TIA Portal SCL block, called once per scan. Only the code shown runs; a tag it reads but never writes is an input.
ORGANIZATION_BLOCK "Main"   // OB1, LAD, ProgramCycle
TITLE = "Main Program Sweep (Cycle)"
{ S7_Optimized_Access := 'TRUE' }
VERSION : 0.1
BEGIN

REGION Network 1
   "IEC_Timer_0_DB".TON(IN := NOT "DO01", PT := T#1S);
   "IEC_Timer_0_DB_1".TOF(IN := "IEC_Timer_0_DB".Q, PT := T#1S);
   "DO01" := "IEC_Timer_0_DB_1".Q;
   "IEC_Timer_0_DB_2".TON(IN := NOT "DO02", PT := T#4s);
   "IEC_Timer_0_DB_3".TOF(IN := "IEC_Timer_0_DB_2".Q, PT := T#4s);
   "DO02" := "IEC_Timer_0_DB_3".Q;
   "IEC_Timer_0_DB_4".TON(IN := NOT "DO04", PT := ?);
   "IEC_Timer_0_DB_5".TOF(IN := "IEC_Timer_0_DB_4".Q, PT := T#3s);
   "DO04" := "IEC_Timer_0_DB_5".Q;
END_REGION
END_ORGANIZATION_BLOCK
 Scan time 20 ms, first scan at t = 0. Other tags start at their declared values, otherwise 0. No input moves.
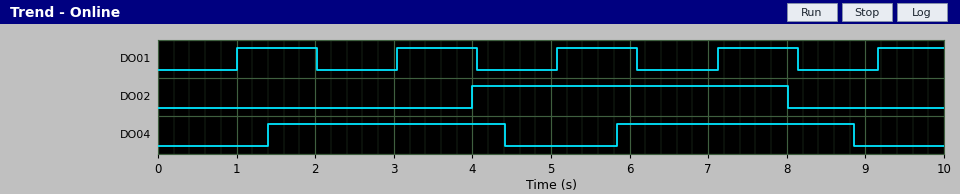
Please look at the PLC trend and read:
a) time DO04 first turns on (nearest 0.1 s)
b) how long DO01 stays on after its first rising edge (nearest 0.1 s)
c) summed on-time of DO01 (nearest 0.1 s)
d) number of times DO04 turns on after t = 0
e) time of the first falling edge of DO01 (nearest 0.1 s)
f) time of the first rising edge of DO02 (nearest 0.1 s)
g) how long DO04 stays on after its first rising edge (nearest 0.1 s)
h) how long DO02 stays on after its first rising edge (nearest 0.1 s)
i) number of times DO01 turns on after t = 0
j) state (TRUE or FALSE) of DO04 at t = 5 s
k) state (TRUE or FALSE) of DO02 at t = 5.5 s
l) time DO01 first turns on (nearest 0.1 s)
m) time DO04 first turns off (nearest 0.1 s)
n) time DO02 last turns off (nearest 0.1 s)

1.4 s
1.0 s
4.9 s
2
2.0 s
4.0 s
3.0 s
4.0 s
5
FALSE
TRUE
1.0 s
4.4 s
8.0 s
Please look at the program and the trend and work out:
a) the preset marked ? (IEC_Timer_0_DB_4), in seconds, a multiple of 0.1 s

1.4 s
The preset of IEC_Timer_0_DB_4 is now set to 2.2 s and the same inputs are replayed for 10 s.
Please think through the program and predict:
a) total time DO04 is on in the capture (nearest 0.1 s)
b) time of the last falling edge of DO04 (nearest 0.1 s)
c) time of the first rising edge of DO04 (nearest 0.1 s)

5.6 s
5.2 s
2.2 s
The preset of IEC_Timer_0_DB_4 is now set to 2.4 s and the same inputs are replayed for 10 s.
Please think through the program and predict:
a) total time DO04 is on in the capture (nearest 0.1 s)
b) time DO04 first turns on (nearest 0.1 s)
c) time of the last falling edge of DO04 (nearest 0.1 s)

5.2 s
2.4 s
5.4 s
